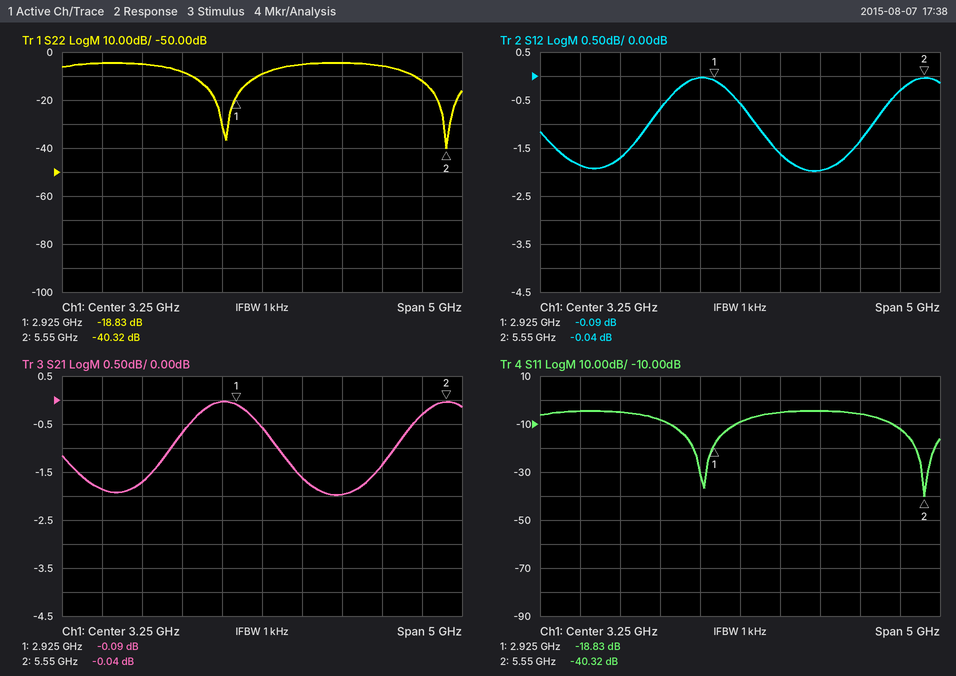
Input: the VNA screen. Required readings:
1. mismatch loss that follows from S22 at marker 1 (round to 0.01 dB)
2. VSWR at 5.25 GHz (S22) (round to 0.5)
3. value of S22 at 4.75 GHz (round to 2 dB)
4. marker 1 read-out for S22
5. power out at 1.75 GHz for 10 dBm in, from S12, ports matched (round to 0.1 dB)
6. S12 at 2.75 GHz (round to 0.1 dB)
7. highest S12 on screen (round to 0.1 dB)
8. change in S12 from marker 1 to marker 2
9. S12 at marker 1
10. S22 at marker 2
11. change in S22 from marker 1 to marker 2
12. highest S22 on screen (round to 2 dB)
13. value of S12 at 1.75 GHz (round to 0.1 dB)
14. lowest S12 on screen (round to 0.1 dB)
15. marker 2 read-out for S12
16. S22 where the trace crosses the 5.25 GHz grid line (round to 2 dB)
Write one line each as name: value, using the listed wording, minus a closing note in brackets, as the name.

mismatch loss that follows from S22 at marker 1: 0.06 dB
VSWR at 5.25 GHz (S22): 1.5
value of S22 at 4.75 GHz: -6 dB
marker 1 read-out for S22: -18.83 dB
power out at 1.75 GHz for 10 dBm in, from S12, ports matched: 8.3 dBm
S12 at 2.75 GHz: 0.0 dB
highest S12 on screen: 0.0 dB
change in S12 from marker 1 to marker 2: 0.05 dB
S12 at marker 1: -0.09 dB
S22 at marker 2: -40.32 dB
change in S22 from marker 1 to marker 2: -21.49 dB
highest S22 on screen: -4 dB
value of S12 at 1.75 GHz: -1.7 dB
lowest S12 on screen: -2.0 dB
marker 2 read-out for S12: -0.04 dB
S22 where the trace crosses the 5.25 GHz grid line: -12 dB
